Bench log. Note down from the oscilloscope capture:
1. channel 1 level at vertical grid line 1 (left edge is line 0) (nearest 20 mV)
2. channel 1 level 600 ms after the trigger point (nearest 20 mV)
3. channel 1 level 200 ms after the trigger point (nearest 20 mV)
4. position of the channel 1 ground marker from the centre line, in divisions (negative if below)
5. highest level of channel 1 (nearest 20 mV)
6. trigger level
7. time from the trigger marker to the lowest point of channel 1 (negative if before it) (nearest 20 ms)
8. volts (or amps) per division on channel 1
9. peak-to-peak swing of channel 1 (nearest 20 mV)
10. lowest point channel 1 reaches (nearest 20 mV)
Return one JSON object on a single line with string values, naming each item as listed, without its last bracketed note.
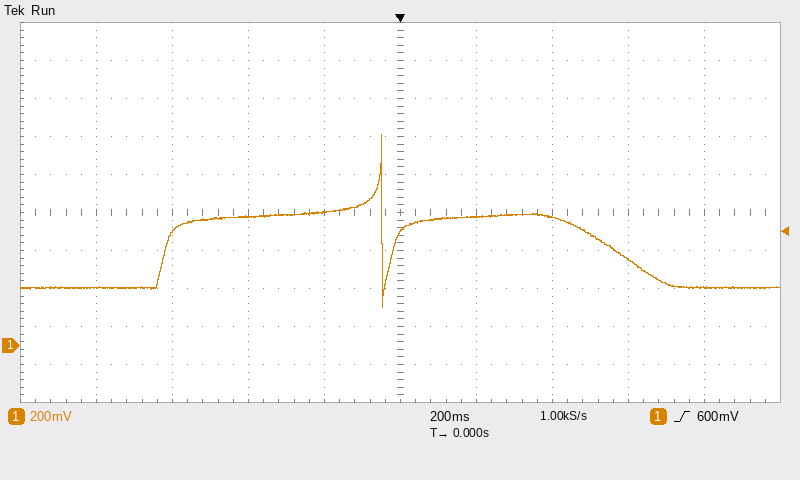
{"channel 1 level at vertical grid line 1 (left edge is line 0)": "300 mV", "channel 1 level 600 ms after the trigger point": "460 mV", "channel 1 level 200 ms after the trigger point": "680 mV", "position of the channel 1 ground marker from the centre line, in divisions": "-3.5 div", "highest level of channel 1": "1.12 V", "trigger level": "600 mV", "time from the trigger marker to the lowest point of channel 1 (negative if before it)": "-40 ms", "volts (or amps) per division on channel 1": "200 mV", "peak-to-peak swing of channel 1": "920 mV", "lowest point channel 1 reaches": "200 mV"}
